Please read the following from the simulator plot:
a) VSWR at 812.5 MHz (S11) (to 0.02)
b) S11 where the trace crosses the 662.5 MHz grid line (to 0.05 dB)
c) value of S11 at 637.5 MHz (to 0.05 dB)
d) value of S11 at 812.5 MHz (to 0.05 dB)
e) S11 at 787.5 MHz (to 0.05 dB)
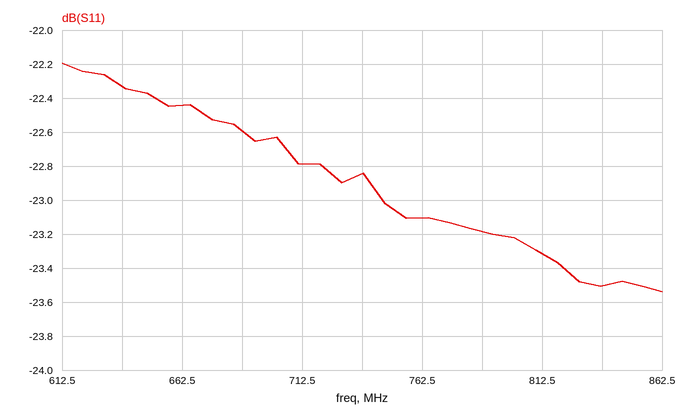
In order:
1.14
-22.45 dB
-22.35 dB
-23.30 dB
-23.20 dB
